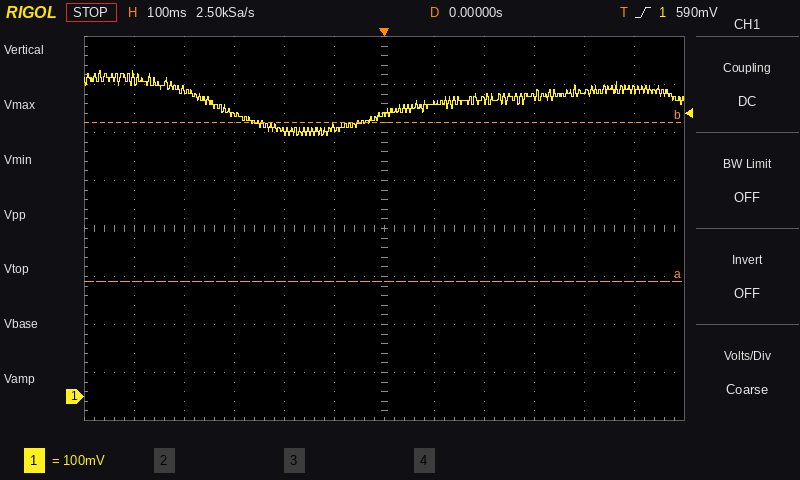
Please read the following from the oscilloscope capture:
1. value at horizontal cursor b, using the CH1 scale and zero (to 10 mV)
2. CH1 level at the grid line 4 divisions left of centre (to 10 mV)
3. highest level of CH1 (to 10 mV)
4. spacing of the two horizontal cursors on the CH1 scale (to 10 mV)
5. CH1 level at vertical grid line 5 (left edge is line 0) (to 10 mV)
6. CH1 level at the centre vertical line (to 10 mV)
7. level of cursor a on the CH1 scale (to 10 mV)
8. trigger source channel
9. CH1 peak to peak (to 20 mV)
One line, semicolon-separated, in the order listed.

570 mV; 640 mV; 680 mV; 330 mV; 560 mV; 590 mV; 240 mV; CH1; 140 mV
